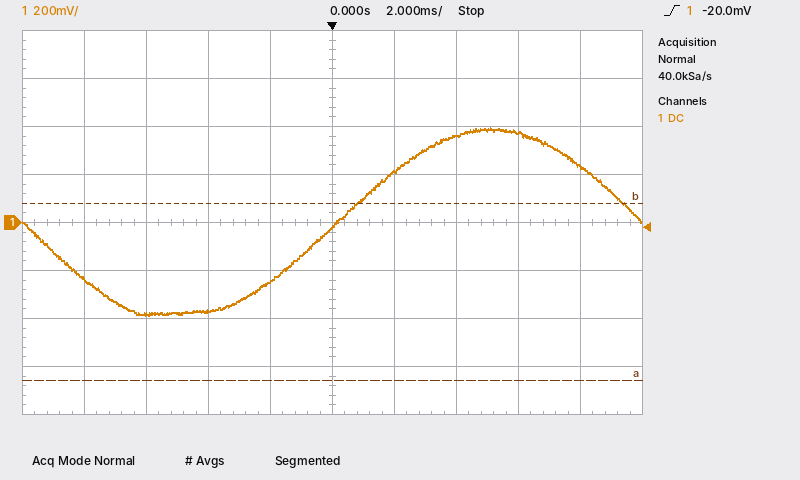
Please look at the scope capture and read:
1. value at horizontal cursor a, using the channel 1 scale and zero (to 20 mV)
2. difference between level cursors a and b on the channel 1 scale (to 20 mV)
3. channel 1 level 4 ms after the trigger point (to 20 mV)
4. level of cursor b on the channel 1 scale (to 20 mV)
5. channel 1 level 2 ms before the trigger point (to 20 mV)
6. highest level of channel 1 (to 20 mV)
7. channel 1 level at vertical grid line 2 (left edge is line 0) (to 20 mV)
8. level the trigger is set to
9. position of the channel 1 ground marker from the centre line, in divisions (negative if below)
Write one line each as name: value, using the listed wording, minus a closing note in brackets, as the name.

value at horizontal cursor a, using the channel 1 scale and zero: -660 mV
difference between level cursors a and b on the channel 1 scale: 740 mV
channel 1 level 4 ms after the trigger point: 360 mV
level of cursor b on the channel 1 scale: 80 mV
channel 1 level 2 ms before the trigger point: -240 mV
highest level of channel 1: 400 mV
channel 1 level at vertical grid line 2 (left edge is line 0): -380 mV
level the trigger is set to: -20.0 mV
position of the channel 1 ground marker from the centre line, in divisions: 0.0 div
